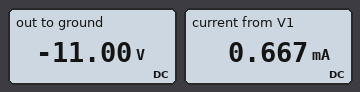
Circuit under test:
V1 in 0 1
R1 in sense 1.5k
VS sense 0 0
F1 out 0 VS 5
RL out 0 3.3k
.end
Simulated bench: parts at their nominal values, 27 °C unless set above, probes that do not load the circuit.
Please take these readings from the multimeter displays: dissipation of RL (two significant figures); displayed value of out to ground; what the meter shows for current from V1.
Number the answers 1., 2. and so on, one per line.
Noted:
1. 37 mW
2. -11.00 V
3. 0.667 mA
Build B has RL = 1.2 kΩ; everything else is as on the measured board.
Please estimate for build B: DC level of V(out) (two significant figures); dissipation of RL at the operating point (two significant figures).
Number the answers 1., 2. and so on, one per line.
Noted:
1. -4.0 V
2. 13 mW
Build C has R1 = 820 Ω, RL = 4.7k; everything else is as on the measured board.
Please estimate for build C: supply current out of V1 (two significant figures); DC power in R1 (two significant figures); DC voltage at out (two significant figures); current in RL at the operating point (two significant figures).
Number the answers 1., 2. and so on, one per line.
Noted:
1. 1.2 mA
2. 1.2 mW
3. -29 V
4. 6.1 mA
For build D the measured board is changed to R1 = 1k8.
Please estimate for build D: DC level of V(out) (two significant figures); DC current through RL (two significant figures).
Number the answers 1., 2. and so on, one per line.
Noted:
1. -9.2 V
2. 2.8 mA
